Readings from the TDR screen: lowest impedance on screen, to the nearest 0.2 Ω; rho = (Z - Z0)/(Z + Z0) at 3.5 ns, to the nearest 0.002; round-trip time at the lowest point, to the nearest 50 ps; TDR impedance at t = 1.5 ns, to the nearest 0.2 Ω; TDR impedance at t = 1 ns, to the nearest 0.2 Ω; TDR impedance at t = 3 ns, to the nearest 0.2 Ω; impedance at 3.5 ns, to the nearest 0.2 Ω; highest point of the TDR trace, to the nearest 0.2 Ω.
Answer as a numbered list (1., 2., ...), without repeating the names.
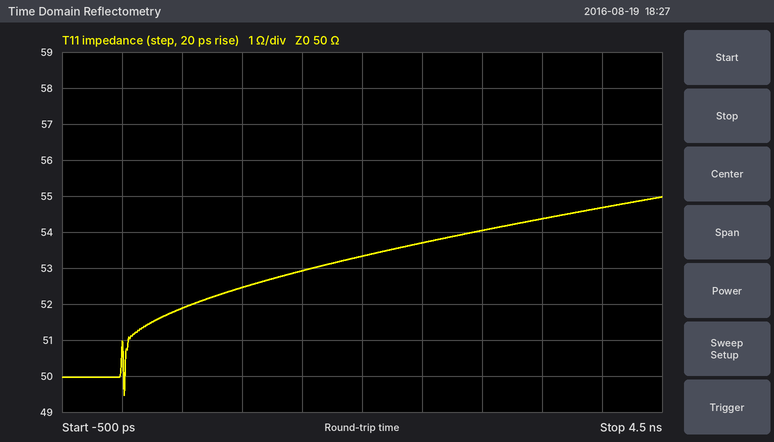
1. 49.4 Ω
2. +0.042
3. 0 ps
4. 53.0 Ω
5. 52.4 Ω
6. 54.0 Ω
7. 54.4 Ω
8. 55.0 Ω
